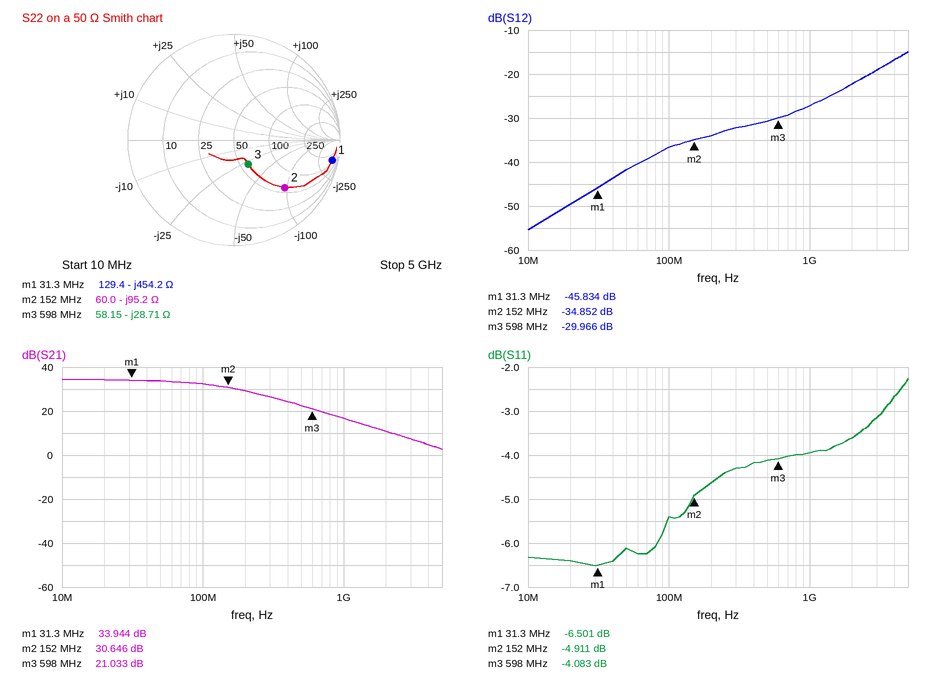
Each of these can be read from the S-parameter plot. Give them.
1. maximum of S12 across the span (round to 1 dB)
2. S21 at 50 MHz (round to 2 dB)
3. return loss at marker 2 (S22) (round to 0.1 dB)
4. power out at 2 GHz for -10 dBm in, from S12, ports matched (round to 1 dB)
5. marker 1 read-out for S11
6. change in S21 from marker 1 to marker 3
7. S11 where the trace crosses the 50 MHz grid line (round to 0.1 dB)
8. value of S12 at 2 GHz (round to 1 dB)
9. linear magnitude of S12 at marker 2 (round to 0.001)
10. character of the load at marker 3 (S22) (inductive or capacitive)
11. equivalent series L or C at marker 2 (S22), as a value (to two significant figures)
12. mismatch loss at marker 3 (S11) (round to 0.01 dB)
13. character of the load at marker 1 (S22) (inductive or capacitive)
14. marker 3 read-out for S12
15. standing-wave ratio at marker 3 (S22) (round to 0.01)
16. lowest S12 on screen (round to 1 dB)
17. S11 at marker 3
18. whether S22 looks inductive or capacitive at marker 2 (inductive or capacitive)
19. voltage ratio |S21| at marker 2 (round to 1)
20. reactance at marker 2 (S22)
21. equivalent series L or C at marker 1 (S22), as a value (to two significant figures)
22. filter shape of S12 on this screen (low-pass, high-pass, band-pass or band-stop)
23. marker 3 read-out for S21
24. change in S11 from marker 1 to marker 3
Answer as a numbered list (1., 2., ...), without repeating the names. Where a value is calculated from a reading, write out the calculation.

1. -15 dB
2. 34 dB
3. 3.6 dB
4. -10 dBm + (-22 dB) = -32 dBm
5. -6.501 dB
6. 21.033 − (33.944) = -12.911 dB
7. -6.1 dB
8. -22 dB
9. 10^(-34.852/20) ≈ 0.018
10. capacitive
11. C = 1/(2π × 152 MHz × 95.2 Ω) ≈ 11 pF
12. −10 log10(1 − 10^(-4.083/10)) ≈ 2.15 dB
13. capacitive
14. -29.966 dB
15. 1.73
16. -55 dB
17. -4.083 dB
18. capacitive
19. 10^(30.646/20) ≈ 34
20. -95.2 Ω
21. C = 1/(2π × 31.3 MHz × 454.2 Ω) ≈ 11 pF
22. high-pass
23. 21.033 dB
24. -4.083 − (-6.501) = 2.418 dB
